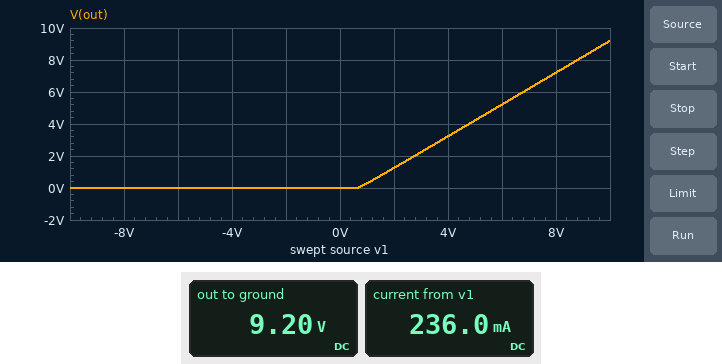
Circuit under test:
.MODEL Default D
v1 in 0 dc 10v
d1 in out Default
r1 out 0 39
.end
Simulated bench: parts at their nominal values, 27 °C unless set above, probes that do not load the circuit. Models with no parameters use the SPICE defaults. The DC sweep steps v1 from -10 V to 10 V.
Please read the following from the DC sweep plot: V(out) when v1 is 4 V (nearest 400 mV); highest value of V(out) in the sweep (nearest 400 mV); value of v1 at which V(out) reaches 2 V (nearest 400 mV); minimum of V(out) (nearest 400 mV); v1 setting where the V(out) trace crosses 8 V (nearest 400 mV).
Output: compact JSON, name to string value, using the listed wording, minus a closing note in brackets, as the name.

{"V(out) when v1 is 4 V": "3.2 V", "highest value of V(out) in the sweep": "9.2 V", "value of v1 at which V(out) reaches 2 V": "2.8 V", "minimum of V(out)": "0 V", "v1 setting where the V(out) trace crosses 8 V": "8.8 V"}
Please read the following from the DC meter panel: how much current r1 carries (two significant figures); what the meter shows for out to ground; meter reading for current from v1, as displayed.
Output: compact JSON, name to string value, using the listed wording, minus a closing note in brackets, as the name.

{"how much current r1 carries": "240 mA", "what the meter shows for out to ground": "9.20 V", "meter reading for current from v1, as displayed": "236.0 mA"}
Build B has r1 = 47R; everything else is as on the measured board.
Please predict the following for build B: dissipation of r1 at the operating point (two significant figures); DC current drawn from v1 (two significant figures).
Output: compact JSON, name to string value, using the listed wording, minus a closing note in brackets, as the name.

{"dissipation of r1 at the operating point": "1.8 W", "DC current drawn from v1": "200 mA"}
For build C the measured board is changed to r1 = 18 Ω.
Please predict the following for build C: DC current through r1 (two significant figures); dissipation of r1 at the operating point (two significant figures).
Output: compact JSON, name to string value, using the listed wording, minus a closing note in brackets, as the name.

{"DC current through r1": "510 mA", "dissipation of r1 at the operating point": "4.7 W"}
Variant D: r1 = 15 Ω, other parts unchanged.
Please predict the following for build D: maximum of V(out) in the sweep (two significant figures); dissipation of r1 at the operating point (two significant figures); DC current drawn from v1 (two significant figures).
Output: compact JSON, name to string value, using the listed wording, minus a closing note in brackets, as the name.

{"maximum of V(out) in the sweep": "9.2 V", "dissipation of r1 at the operating point": "5.6 W", "DC current drawn from v1": "610 mA"}
